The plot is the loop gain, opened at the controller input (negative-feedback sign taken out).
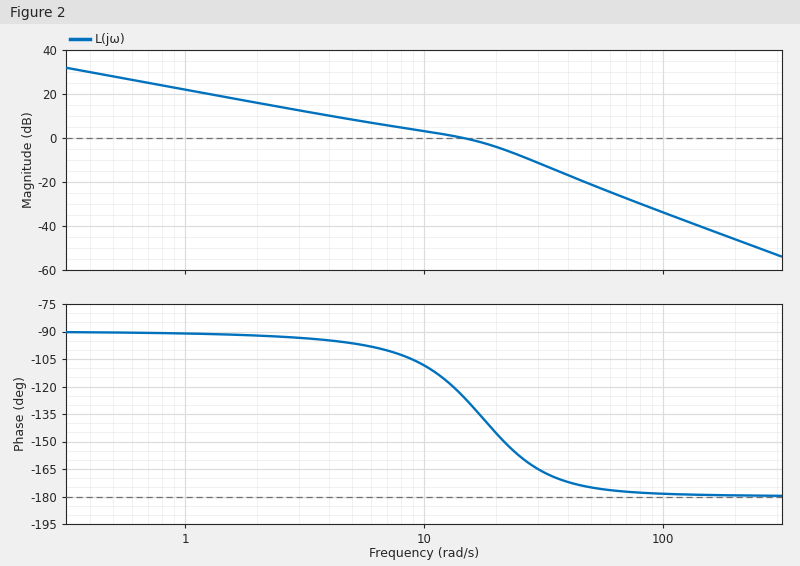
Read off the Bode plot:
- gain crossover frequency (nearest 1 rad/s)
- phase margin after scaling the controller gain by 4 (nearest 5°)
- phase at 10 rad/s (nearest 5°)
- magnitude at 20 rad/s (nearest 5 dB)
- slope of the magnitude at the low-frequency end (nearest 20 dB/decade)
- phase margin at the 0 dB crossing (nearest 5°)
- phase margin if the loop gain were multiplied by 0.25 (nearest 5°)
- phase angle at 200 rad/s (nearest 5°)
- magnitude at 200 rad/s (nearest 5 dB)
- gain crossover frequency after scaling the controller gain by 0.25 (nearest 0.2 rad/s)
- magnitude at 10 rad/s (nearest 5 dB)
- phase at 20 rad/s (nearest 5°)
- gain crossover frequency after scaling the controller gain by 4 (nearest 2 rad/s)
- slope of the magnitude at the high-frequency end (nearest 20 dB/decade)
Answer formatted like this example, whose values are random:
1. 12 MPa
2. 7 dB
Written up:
1. 15 rad/s
2. 15°
3. -110°
4. -5 dB
5. -20 dB/decade
6. 55°
7. 85°
8. -180°
9. -45 dB
10. 3.2 rad/s
11. 5 dB
12. -145°
13. 32 rad/s
14. -40 dB/decade
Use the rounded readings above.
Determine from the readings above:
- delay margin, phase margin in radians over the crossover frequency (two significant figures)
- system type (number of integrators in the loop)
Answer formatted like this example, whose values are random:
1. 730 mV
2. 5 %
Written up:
1. 0.064 s
2. 1
